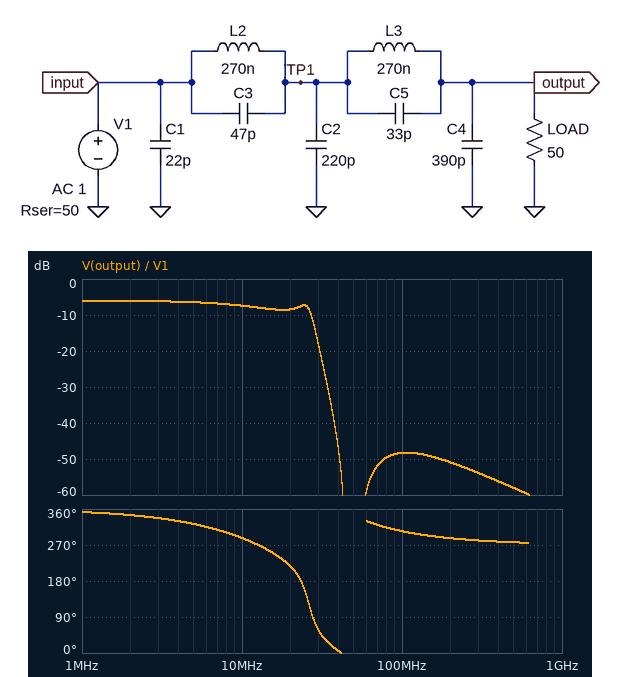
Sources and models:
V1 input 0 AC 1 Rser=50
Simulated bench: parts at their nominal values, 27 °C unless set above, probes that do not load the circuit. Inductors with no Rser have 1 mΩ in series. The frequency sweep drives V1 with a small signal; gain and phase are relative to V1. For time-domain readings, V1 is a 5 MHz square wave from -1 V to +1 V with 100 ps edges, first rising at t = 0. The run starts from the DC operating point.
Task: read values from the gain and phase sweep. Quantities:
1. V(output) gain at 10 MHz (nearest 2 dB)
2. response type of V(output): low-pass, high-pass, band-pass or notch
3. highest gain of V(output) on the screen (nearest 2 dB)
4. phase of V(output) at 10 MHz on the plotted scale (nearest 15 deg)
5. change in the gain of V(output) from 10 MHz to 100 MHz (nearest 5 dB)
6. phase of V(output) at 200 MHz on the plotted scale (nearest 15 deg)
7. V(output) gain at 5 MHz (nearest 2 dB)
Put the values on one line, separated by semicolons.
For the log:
-8 dB; low-pass; -6 dB; 285 deg; -40 dB; 285 deg; -6 dB
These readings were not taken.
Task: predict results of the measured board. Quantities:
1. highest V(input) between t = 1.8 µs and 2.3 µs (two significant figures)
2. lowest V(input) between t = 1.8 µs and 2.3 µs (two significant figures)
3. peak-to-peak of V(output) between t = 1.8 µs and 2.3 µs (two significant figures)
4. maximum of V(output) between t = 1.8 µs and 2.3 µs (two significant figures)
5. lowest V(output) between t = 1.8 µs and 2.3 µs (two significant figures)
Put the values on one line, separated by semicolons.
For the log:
780 mV; -780 mV; 1.1 V; 560 mV; -560 mV
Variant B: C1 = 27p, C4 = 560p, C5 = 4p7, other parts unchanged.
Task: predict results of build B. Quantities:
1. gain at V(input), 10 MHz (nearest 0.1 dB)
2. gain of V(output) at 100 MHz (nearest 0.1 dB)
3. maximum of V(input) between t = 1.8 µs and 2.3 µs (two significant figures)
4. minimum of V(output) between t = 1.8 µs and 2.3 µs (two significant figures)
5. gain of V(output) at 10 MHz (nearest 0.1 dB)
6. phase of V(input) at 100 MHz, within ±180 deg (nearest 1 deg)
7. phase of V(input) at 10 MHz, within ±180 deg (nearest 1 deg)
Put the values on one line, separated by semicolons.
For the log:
-11.6 dB; -64.5 dB; 820 mV; -530 mV; -8.5 dB; -62 deg; 36 deg
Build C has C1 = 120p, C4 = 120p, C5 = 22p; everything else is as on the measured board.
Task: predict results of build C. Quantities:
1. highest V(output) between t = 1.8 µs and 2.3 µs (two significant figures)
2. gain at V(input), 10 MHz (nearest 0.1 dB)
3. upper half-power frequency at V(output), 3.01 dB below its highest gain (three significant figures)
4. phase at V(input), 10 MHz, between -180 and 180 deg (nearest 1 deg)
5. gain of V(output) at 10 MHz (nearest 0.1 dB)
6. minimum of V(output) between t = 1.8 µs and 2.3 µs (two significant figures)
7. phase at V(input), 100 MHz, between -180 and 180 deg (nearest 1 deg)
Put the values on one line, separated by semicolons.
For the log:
650 mV; -8.2 dB; 30.5 MHz; -10 deg; -6.3 dB; -650 mV; -78 deg
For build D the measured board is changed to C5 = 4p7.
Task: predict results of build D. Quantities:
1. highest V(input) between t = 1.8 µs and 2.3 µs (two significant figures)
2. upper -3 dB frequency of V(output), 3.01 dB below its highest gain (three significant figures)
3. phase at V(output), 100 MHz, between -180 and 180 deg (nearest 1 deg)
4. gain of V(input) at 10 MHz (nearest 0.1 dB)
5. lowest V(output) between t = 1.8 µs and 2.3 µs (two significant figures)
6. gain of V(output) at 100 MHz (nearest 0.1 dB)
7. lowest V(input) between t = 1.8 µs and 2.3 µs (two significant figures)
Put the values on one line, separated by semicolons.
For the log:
870 mV; 29.5 MHz; 125 deg; -11.7 dB; -550 mV; -60.8 dB; -870 mV
